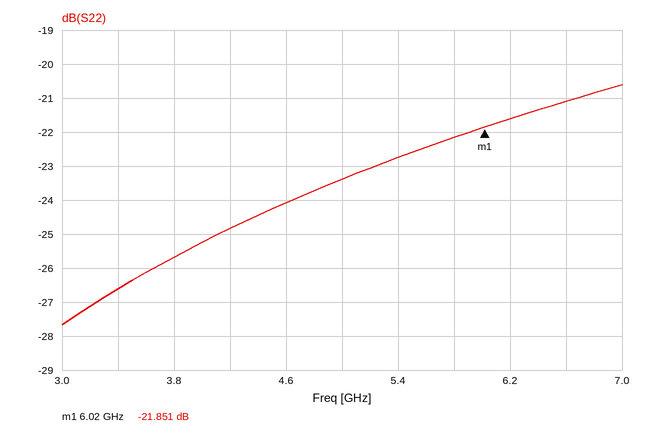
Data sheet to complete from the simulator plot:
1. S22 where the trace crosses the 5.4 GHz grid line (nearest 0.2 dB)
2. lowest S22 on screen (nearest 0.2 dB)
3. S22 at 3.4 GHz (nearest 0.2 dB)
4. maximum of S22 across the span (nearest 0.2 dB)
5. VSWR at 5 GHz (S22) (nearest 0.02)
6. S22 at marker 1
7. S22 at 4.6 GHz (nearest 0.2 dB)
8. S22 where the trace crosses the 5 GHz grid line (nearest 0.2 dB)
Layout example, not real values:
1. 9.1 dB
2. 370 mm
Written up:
1. -22.8 dB
2. -27.6 dB
3. -26.6 dB
4. -20.6 dB
5. 1.14
6. -21.851 dB
7. -24.0 dB
8. -23.4 dB
